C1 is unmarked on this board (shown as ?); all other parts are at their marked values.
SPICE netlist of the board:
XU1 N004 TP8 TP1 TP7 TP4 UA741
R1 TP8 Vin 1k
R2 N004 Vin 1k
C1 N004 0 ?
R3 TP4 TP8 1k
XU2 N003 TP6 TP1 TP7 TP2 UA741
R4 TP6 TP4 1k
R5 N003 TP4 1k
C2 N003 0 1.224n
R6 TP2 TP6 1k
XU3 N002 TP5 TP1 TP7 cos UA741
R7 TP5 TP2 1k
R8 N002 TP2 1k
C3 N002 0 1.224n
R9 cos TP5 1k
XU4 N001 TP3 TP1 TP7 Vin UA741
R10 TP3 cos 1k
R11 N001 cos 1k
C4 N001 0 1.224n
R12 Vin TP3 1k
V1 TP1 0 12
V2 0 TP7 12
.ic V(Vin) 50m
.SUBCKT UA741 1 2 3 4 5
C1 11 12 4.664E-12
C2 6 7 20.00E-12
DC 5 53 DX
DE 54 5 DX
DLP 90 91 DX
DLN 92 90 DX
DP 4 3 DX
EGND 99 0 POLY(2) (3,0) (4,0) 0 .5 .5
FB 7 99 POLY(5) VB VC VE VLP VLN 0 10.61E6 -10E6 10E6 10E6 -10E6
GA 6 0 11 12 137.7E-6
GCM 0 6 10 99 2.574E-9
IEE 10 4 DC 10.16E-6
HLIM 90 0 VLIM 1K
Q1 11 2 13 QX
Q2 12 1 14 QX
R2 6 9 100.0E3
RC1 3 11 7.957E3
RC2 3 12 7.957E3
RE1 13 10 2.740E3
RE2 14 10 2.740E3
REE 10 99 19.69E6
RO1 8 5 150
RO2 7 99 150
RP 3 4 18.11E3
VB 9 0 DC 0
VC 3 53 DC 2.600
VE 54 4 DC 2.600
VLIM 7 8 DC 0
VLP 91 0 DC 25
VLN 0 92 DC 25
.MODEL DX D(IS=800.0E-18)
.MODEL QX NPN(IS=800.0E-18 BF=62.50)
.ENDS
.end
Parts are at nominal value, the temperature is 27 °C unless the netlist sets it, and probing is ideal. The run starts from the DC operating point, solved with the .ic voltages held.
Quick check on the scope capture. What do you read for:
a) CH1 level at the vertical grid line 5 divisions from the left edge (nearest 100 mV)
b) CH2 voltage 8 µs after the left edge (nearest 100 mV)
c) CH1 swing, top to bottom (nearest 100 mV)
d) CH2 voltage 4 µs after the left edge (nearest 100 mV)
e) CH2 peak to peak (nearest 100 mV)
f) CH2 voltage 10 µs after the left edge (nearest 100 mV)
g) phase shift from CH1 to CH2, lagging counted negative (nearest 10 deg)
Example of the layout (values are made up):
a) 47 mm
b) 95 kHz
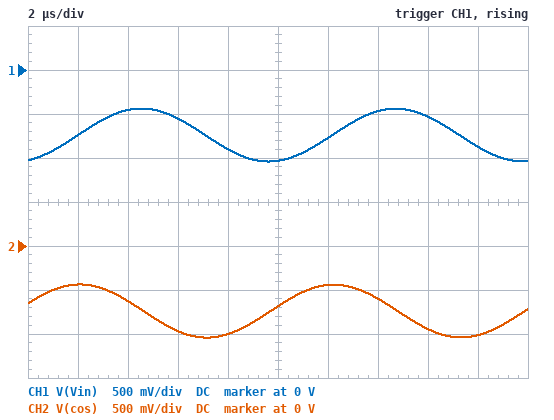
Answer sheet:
a) -1.0 V
b) -1.0 V
c) 600 mV
d) -600 mV
e) 600 mV
f) -700 mV
g) 90 deg
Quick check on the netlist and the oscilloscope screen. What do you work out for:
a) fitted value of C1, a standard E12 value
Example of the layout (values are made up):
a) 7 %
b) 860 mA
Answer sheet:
a) 1.5 nF
